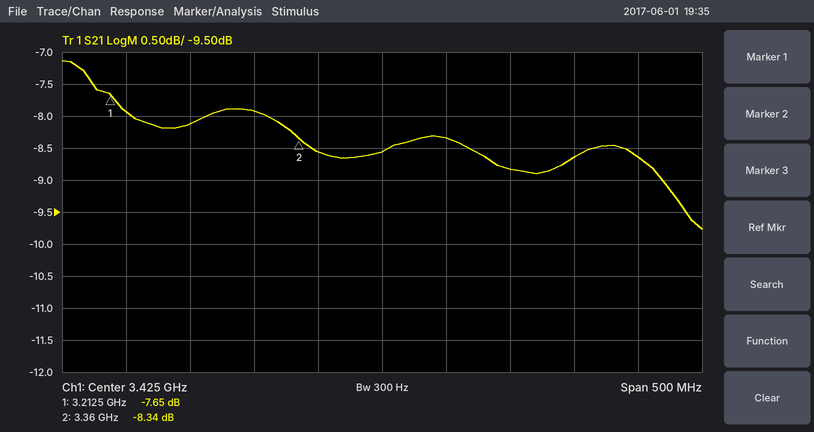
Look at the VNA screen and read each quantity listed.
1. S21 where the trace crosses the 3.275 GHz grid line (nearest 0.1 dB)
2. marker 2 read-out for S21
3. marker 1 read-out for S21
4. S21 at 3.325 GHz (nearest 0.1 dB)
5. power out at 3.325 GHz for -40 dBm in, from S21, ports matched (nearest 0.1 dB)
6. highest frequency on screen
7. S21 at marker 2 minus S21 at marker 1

-8.1 dB
-8.34 dB
-7.65 dB
-7.9 dB
-47.9 dBm
3.675 GHz
-0.69 dB
